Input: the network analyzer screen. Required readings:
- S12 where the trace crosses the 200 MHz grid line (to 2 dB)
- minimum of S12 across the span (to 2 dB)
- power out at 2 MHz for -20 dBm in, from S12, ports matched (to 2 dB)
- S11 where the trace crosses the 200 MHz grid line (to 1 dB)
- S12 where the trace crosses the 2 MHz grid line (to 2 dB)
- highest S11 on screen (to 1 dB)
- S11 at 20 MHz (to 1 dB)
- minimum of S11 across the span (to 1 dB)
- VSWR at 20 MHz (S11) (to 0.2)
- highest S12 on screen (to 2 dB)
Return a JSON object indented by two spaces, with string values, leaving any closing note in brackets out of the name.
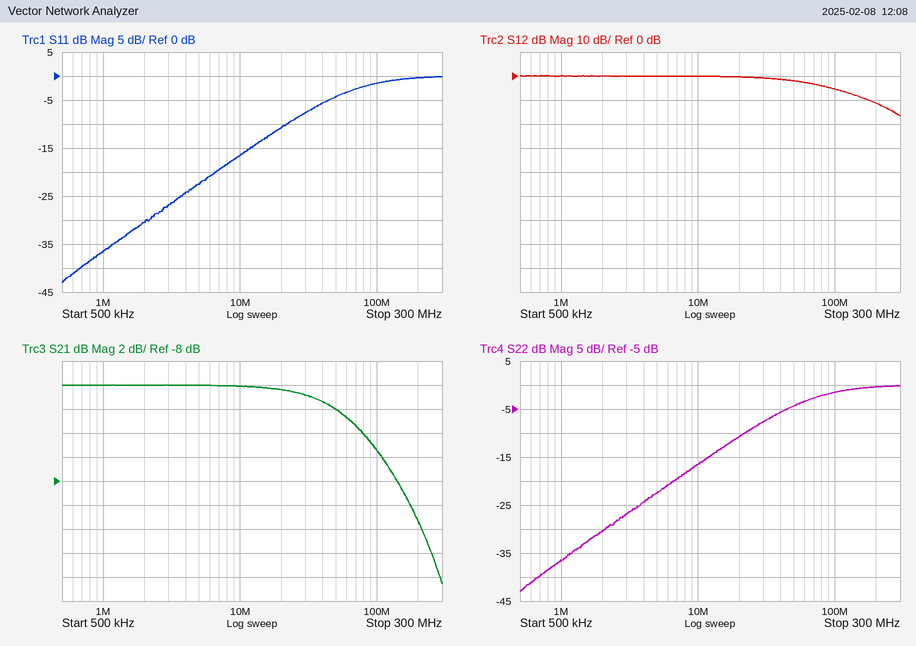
{
  "S12 where the trace crosses the 200 MHz grid line": "-12 dB",
  "minimum of S12 across the span": "-16 dB",
  "power out at 2 MHz for -20 dBm in, from S12, ports matched": "-20 dBm",
  "S11 where the trace crosses the 200 MHz grid line": "0 dB",
  "S12 where the trace crosses the 2 MHz grid line": "0 dB",
  "highest S11 on screen": "0 dB",
  "S11 at 20 MHz": "-11 dB",
  "minimum of S11 across the span": "-43 dB",
  "VSWR at 20 MHz (S11)": "1.8",
  "highest S12 on screen": "0 dB"
}
